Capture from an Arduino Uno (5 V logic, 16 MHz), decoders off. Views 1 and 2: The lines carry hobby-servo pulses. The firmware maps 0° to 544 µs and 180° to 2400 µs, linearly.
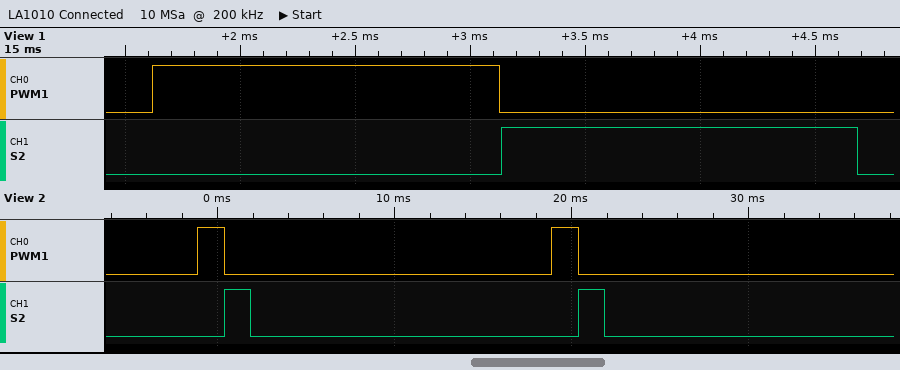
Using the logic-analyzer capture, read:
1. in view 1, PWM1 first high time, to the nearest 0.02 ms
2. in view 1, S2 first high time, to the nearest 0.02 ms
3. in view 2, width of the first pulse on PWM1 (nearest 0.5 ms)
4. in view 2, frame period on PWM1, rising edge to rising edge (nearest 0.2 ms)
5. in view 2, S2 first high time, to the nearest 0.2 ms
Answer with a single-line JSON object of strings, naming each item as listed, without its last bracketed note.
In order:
{"in view 1, PWM1 first high time, to the nearest 0.02 ms": "1.50 ms", "in view 1, S2 first high time, to the nearest 0.02 ms": "1.54 ms", "in view 2, width of the first pulse on PWM1": "1.5 ms", "in view 2, frame period on PWM1, rising edge to rising edge": "20.0 ms", "in view 2, S2 first high time, to the nearest 0.2 ms": "1.4 ms"}
